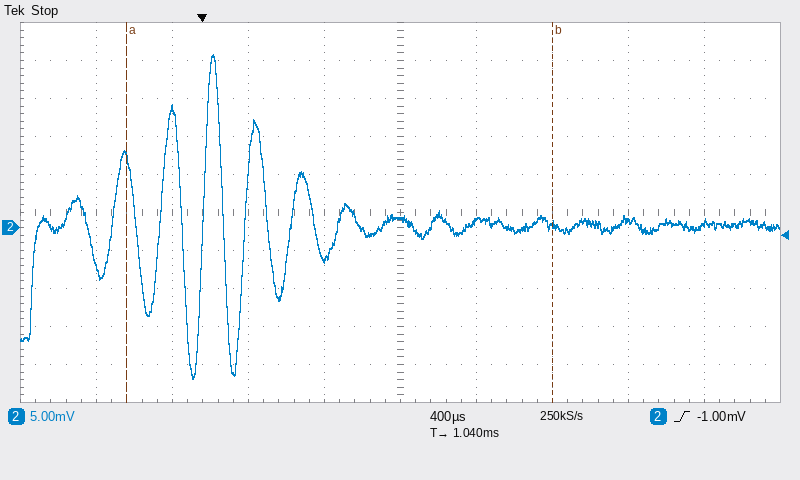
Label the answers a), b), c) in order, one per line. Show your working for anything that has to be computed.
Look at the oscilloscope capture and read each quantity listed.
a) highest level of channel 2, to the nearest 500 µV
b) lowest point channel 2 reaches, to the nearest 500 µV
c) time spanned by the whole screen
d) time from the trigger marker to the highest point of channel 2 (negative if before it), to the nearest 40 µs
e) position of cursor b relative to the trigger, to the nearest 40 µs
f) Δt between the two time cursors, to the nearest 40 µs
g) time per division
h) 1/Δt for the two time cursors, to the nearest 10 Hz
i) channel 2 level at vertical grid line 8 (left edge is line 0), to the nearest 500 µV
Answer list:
a) 23.0 mV
b) -20.0 mV
c) 4 ms
d) +40 µs
e) +1.84 ms
f) 2.24 ms
g) 400 µs
h) 1 / 2.24 ms ≈ 450 Hz
i) 1.0 mV
